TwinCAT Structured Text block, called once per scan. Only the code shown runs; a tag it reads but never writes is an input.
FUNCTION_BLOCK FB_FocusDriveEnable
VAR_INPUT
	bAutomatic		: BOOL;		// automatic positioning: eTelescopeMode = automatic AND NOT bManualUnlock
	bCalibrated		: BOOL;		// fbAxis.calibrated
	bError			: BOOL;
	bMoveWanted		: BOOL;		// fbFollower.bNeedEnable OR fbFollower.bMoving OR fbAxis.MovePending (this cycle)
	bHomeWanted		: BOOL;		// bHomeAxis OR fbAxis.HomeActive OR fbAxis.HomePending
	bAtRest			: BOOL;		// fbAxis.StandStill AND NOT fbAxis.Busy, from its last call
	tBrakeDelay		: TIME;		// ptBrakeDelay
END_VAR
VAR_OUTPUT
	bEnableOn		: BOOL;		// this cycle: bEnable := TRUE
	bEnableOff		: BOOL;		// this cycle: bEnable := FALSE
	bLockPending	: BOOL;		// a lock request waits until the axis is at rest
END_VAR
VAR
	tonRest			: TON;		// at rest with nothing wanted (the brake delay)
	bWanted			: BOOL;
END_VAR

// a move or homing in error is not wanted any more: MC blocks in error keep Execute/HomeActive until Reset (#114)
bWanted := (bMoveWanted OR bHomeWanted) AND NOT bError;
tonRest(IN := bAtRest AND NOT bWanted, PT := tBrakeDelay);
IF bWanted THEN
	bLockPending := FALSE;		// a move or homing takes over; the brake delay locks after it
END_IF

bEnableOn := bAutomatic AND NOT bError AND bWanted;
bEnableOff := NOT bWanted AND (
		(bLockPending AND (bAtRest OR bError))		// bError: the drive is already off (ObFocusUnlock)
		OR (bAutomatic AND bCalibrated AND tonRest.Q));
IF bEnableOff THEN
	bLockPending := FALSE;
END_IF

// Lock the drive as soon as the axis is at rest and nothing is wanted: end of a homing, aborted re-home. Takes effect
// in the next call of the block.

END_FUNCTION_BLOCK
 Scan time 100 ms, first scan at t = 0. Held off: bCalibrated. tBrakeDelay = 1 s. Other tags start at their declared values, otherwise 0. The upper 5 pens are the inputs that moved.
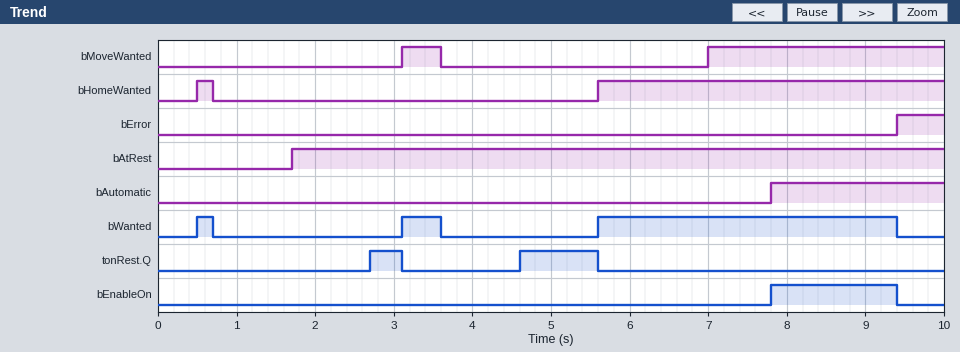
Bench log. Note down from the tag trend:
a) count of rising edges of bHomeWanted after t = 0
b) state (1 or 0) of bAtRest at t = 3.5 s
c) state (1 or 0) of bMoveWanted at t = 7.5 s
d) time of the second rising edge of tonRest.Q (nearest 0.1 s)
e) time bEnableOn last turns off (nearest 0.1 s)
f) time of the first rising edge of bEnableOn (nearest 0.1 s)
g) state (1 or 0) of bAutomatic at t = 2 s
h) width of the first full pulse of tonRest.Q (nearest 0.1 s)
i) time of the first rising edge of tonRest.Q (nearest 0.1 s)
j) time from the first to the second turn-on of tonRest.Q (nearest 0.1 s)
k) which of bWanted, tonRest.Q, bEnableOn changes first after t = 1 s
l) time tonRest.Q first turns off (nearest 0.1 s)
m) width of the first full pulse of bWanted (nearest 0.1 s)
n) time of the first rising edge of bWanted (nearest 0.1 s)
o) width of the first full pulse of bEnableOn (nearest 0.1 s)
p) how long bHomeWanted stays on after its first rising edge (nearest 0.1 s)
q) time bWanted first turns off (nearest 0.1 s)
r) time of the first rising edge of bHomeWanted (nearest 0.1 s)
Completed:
2
1
1
4.6 s
9.4 s
7.8 s
0
0.4 s
2.7 s
1.9 s
tonRest.Q
3.1 s
0.2 s
0.5 s
1.6 s
0.2 s
0.7 s
0.5 s
